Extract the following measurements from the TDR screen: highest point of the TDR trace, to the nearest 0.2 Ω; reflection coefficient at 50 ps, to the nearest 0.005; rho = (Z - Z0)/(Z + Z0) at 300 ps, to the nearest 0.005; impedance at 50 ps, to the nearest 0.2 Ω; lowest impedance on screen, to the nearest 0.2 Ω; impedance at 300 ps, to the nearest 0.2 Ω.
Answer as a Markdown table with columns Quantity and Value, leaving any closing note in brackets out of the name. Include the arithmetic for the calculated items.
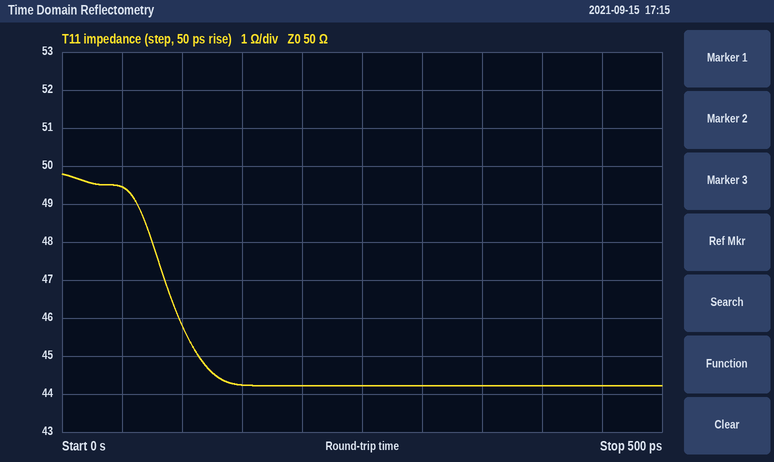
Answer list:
| Quantity | Value |
|---|---|
| highest point of the TDR trace, to the nearest 0.2 Ω | 49.8 Ω |
| reflection coefficient at 50 ps, to the nearest 0.005 | (49.4 − 50)/(49.4 + 50) ≈ -0.00604, so -0.005 to the nearest 0.005 |
| rho = (Z - Z0)/(Z + Z0) at 300 ps, to the nearest 0.005 | (44.2 − 50)/(44.2 + 50) ≈ -0.0616, so -0.060 to the nearest 0.005 |
| impedance at 50 ps, to the nearest 0.2 Ω | 49.4 Ω |
| lowest impedance on screen, to the nearest 0.2 Ω | 44.2 Ω |
| impedance at 300 ps, to the nearest 0.2 Ω | 44.2 Ω |
